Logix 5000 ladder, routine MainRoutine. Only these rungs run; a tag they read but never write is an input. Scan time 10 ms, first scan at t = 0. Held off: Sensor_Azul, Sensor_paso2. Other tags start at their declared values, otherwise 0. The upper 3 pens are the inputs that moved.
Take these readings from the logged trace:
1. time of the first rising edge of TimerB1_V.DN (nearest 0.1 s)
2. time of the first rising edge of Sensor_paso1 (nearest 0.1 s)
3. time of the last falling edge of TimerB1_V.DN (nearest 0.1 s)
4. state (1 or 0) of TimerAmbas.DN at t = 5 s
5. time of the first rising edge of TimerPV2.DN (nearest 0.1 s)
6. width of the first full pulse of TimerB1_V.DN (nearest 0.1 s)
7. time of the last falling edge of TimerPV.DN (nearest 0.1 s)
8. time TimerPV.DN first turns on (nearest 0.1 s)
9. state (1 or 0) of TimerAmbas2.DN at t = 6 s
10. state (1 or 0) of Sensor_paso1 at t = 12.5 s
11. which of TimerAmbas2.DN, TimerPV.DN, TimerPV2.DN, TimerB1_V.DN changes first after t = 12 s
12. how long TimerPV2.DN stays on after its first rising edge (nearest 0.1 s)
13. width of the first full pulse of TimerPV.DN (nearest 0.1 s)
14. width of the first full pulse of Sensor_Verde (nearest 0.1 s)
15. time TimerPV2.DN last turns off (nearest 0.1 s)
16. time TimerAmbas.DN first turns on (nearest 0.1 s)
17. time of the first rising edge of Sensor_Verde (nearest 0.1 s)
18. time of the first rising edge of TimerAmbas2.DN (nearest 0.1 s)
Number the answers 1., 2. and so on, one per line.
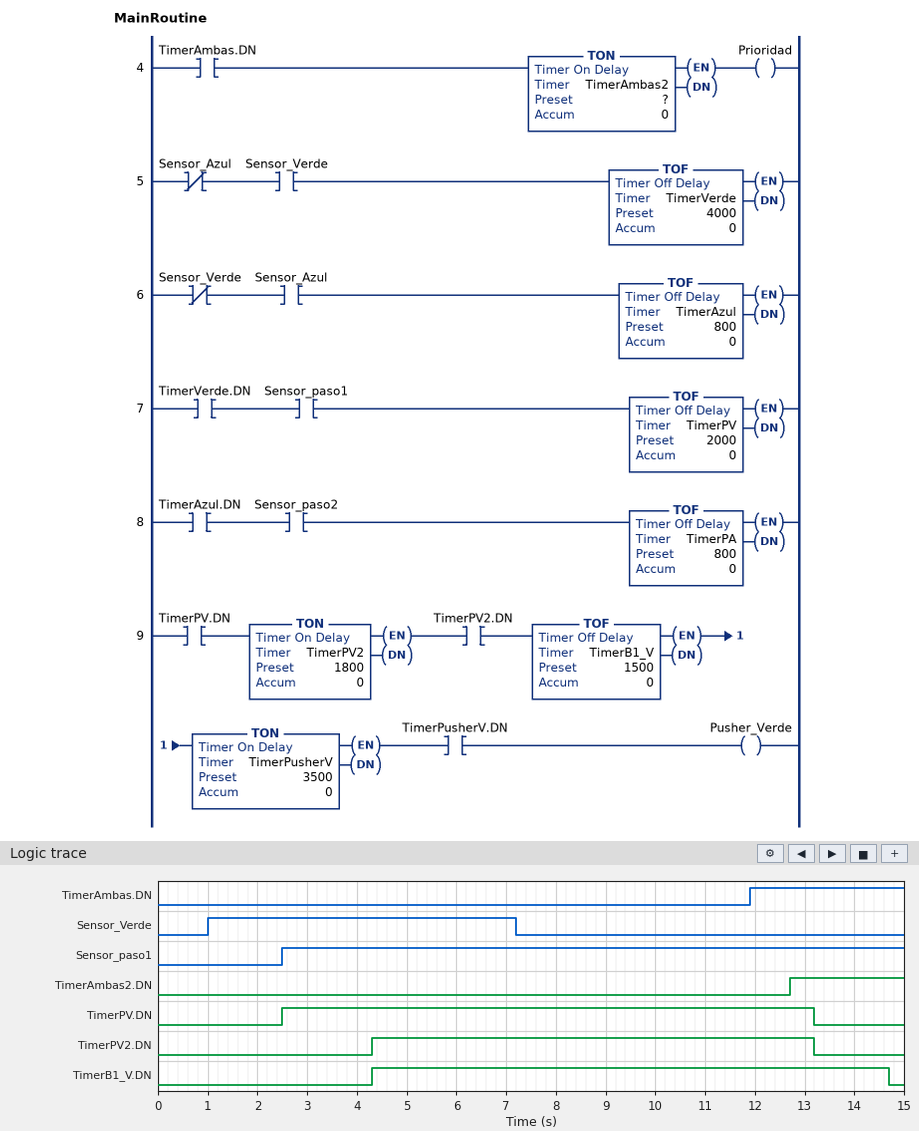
1. 4.3 s
2. 2.5 s
3. 14.7 s
4. 0
5. 4.3 s
6. 10.4 s
7. 13.2 s
8. 2.5 s
9. 0
10. 1
11. TimerAmbas2.DN
12. 8.9 s
13. 10.7 s
14. 6.2 s
15. 13.2 s
16. 11.9 s
17. 1.0 s
18. 12.7 s
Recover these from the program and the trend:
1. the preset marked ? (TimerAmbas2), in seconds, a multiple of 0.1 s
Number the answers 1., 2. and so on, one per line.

1. 0.8 s
